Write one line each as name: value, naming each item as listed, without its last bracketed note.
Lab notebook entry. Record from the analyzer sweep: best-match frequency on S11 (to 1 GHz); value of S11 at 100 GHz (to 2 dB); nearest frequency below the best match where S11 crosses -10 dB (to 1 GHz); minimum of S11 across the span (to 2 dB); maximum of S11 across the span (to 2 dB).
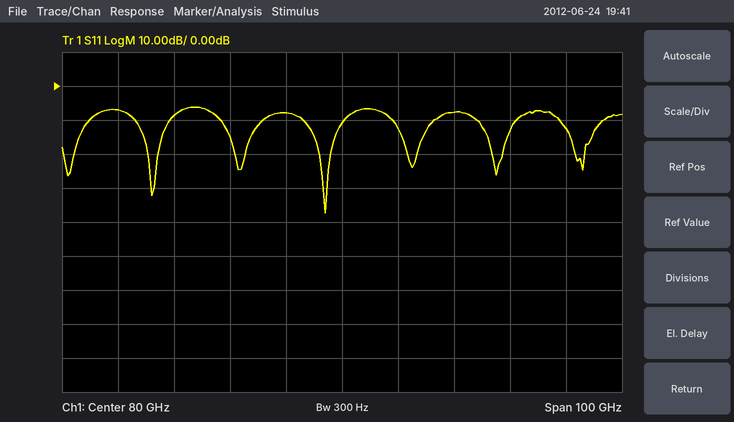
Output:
best-match frequency on S11: 77 GHz
value of S11 at 100 GHz: -8 dB
nearest frequency below the best match where S11 crosses -10 dB: 73 GHz
minimum of S11 across the span: -38 dB
maximum of S11 across the span: -6 dB
